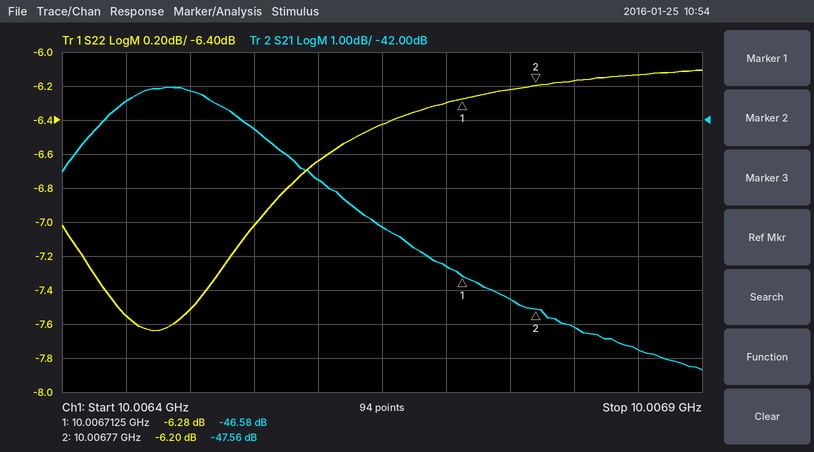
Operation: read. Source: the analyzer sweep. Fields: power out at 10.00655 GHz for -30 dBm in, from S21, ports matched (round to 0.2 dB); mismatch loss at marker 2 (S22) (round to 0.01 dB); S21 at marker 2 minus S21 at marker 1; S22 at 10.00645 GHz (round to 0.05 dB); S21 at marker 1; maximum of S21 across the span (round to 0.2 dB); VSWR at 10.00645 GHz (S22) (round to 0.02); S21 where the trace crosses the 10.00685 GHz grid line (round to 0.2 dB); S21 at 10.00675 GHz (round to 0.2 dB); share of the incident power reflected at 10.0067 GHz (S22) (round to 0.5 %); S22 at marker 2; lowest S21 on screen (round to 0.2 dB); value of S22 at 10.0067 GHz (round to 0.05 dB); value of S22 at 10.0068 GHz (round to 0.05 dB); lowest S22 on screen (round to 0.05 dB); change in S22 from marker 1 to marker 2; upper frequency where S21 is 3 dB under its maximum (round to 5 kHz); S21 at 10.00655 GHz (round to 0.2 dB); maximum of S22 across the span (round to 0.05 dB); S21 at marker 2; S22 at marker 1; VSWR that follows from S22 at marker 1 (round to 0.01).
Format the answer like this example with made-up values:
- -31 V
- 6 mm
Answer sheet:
- -72.2 dBm
- 1.19 dB
- -0.98 dB
- -7.55 dB
- -46.58 dB
- -41.0 dB
- 2.44
- -48.8 dB
- -47.2 dB
- 23.5 %
- -6.20 dB
- -49.4 dB
- -6.30 dB
- -6.15 dB
- -7.65 dB
- 0.08 dB
- 10.006610 GHz
- -42.2 dB
- -6.10 dB
- -47.56 dB
- -6.28 dB
- 2.89
